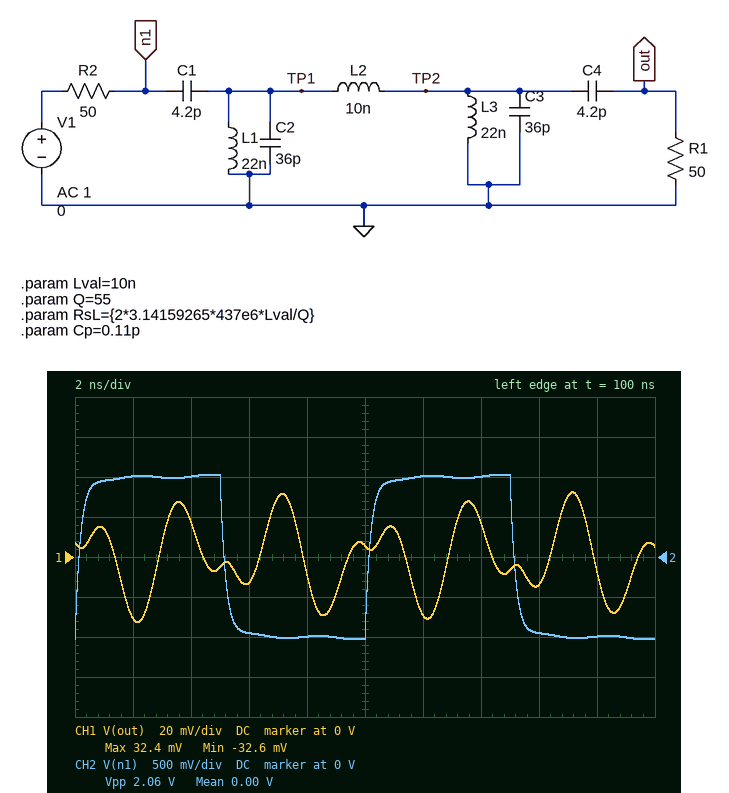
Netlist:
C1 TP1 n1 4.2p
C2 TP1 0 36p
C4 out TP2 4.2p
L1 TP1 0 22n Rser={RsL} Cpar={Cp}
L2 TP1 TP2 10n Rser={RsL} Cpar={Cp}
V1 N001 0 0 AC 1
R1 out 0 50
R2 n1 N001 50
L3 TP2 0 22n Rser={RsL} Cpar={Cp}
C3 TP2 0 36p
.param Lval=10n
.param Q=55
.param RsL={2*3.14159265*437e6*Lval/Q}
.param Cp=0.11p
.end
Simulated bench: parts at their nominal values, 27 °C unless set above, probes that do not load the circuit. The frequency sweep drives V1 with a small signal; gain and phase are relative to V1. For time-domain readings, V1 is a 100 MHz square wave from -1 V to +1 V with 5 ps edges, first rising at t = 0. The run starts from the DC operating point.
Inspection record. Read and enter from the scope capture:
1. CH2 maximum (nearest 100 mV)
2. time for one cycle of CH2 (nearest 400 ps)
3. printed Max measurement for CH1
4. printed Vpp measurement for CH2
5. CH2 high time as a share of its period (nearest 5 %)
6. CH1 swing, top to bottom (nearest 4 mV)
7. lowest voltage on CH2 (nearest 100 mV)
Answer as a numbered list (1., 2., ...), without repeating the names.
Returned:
1. 1.0 V
2. 10.0 ns
3. 32.4 mV
4. 2.06 V
5. 50 %
6. 64 mV
7. -1.0 V
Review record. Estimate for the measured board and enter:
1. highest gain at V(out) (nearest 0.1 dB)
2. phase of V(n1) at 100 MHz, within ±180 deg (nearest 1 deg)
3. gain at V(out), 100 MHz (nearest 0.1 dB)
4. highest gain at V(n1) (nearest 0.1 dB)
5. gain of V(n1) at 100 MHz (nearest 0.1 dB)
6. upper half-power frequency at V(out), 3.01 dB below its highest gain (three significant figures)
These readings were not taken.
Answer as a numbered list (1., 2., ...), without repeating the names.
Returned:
1. -9.0 dB
2. -8 deg
3. -50.0 dB
4. 0 dB
5. -0.1 dB
6. 408 MHz
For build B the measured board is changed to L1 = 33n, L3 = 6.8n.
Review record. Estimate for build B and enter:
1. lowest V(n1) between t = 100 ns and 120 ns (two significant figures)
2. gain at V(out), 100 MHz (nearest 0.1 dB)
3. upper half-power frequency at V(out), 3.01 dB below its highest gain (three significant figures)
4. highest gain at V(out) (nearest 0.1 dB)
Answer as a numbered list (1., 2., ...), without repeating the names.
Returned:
1. -1.0 V
2. -57.6 dB
3. 456 MHz
4. -10.5 dB
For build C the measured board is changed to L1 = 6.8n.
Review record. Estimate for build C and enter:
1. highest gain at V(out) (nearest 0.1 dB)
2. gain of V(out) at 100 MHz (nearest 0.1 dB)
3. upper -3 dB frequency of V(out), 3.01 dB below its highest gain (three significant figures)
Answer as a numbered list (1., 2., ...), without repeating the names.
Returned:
1. -10.2 dB
2. -59.3 dB
3. 459 MHz
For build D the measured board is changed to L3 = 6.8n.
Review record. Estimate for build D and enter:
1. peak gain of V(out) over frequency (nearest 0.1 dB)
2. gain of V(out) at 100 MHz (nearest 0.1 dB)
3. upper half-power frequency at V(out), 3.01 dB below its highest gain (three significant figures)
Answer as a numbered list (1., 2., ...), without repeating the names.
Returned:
1. -10.2 dB
2. -59.3 dB
3. 459 MHz
